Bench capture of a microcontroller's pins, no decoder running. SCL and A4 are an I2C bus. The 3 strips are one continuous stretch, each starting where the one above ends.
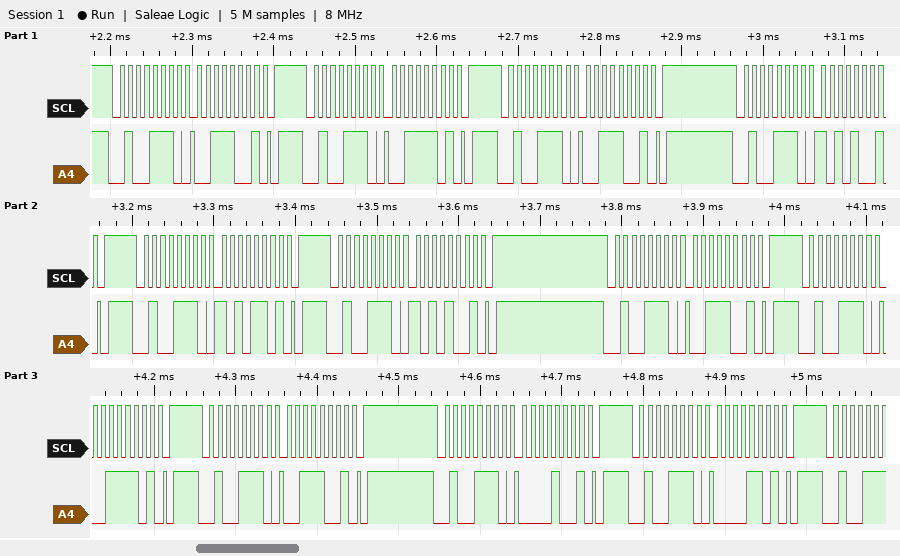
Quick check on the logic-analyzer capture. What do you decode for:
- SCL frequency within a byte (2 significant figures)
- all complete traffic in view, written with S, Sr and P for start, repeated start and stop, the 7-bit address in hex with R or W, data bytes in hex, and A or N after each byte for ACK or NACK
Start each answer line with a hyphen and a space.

- 100 kHz
- S 27W A 39 A P S 27W A 3D A P S 27W A 39 A P S 27W A A9 A P S 27W A AD A P S 27W A A9 A P S 27W A 39 A P S 27W A 3D A P S 27W A 39 A P S 27W A 09 A P S 27W A 0D A P
